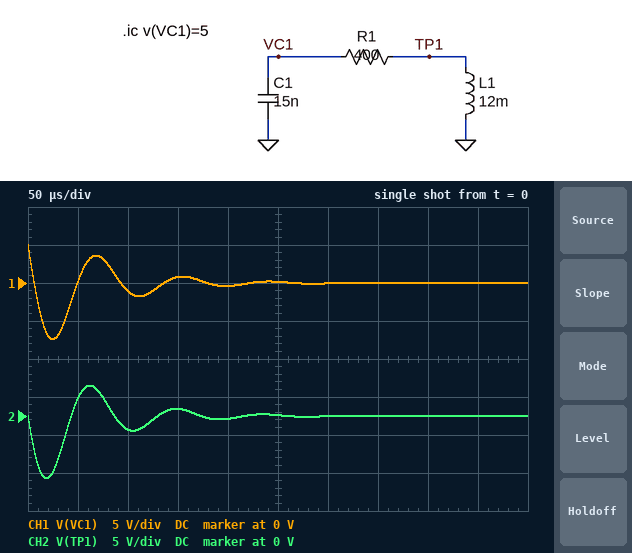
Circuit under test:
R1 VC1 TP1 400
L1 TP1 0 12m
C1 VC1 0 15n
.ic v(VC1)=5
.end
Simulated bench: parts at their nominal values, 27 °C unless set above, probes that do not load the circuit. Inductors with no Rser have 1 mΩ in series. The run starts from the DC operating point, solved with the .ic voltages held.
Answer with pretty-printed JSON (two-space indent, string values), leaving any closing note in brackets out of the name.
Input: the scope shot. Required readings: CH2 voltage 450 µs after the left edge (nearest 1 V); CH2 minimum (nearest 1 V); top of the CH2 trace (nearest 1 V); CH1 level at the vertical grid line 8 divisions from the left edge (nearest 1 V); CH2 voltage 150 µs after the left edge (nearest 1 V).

{
  "CH2 voltage 450 µs after the left edge": "0 V",
  "CH2 minimum": "-8 V",
  "top of the CH2 trace": "4 V",
  "CH1 level at the vertical grid line 8 divisions from the left edge": "0 V",
  "CH2 voltage 150 µs after the left edge": "1 V"
}
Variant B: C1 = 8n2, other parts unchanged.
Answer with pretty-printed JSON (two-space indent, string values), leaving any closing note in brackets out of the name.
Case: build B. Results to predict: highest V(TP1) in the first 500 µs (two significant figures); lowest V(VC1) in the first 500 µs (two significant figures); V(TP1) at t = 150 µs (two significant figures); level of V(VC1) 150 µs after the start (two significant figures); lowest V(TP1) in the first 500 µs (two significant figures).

{
  "highest V(TP1) in the first 500 µs": "7.1 V",
  "lowest V(VC1) in the first 500 µs": "-11 V",
  "V(TP1) at t = 150 µs": "-900 mV",
  "level of V(VC1) 150 µs after the start": "-1.1 V",
  "lowest V(TP1) in the first 500 µs": "-12 V"
}
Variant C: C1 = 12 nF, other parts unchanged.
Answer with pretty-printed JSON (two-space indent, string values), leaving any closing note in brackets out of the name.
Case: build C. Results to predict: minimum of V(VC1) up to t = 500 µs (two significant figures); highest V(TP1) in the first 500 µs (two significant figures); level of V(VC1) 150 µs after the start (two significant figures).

{
  "minimum of V(VC1) up to t = 500 µs": "-8.7 V",
  "highest V(TP1) in the first 500 µs": "5.0 V",
  "level of V(VC1) 150 µs after the start": "690 mV"
}
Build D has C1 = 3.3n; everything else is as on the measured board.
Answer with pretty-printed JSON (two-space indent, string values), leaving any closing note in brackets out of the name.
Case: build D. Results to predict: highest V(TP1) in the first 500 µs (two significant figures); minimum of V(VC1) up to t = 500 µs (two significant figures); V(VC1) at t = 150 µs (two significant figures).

{
  "highest V(TP1) in the first 500 µs": "15 V",
  "minimum of V(VC1) up to t = 500 µs": "-20 V",
  "V(VC1) at t = 150 µs": "2.0 V"
}
